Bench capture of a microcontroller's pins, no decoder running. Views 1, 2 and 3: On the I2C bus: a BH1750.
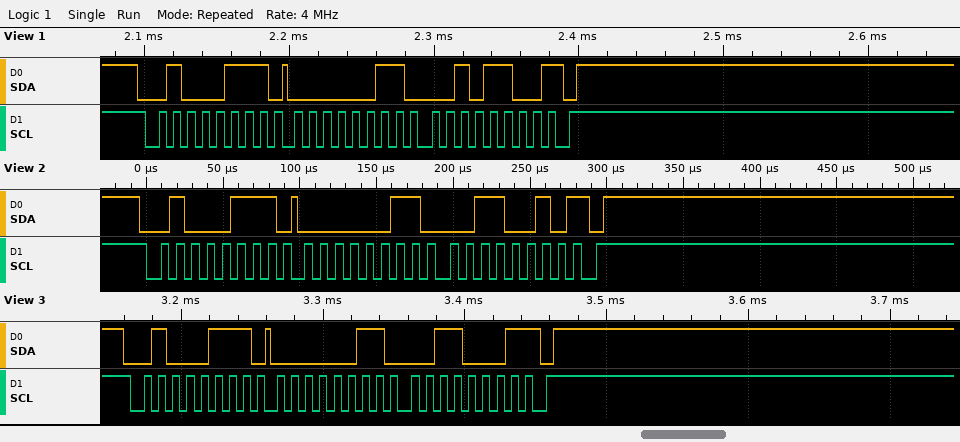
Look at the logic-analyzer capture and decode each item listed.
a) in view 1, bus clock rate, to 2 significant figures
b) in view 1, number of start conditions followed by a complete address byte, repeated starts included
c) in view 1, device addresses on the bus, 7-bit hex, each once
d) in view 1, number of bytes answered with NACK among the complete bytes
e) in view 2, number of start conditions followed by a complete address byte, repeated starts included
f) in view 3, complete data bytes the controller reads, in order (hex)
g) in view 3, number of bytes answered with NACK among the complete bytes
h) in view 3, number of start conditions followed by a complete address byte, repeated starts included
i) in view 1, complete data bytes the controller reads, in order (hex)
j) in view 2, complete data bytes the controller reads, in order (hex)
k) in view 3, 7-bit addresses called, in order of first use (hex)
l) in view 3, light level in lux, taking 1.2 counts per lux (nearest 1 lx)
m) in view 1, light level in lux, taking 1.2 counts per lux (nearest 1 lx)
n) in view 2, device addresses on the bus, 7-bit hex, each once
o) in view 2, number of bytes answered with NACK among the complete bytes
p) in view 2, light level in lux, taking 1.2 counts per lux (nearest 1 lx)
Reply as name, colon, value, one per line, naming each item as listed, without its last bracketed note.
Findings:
in view 1, bus clock rate, to 2 significant figures: 100 kHz
in view 1, number of start conditions followed by a complete address byte, repeated starts included: 1
in view 1, device addresses on the bus, 7-bit hex, each once: 0x23
in view 1, number of bytes answered with NACK among the complete bytes: 1
in view 2, number of start conditions followed by a complete address byte, repeated starts included: 1
in view 3, complete data bytes the controller reads, in order: 03 31
in view 3, number of bytes answered with NACK among the complete bytes: 1
in view 3, number of start conditions followed by a complete address byte, repeated starts included: 1
in view 1, complete data bytes the controller reads, in order: 03 2C
in view 2, complete data bytes the controller reads, in order: 03 32
in view 3, 7-bit addresses called, in order of first use: 0x23
in view 3, light level in lux, taking 1.2 counts per lux: 681 lx
in view 1, light level in lux, taking 1.2 counts per lux: 677 lx
in view 2, device addresses on the bus, 7-bit hex, each once: 0x23
in view 2, number of bytes answered with NACK among the complete bytes: 1
in view 2, light level in lux, taking 1.2 counts per lux: 682 lx
